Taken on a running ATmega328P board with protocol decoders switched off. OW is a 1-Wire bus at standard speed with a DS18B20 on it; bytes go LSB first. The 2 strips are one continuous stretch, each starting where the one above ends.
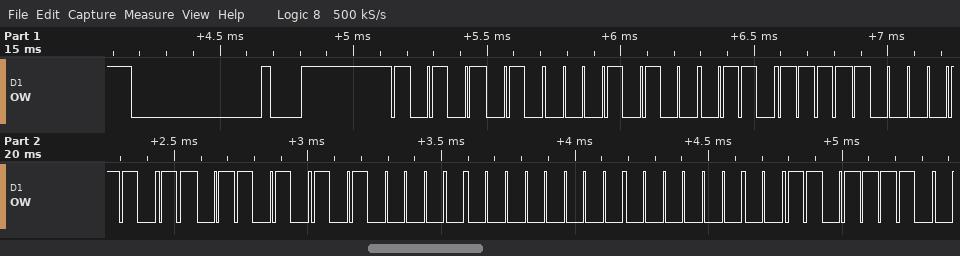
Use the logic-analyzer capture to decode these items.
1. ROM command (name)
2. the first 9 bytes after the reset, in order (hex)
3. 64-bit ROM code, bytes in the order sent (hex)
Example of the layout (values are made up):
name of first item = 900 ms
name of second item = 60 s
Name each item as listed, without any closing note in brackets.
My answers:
ROM command = Match ROM
the first 9 bytes after the reset, in order = 55 28 F6 61 5B 05 00 00 7B
64-bit ROM code, bytes in the order sent = 28 F6 61 5B 05 00 00 7B
